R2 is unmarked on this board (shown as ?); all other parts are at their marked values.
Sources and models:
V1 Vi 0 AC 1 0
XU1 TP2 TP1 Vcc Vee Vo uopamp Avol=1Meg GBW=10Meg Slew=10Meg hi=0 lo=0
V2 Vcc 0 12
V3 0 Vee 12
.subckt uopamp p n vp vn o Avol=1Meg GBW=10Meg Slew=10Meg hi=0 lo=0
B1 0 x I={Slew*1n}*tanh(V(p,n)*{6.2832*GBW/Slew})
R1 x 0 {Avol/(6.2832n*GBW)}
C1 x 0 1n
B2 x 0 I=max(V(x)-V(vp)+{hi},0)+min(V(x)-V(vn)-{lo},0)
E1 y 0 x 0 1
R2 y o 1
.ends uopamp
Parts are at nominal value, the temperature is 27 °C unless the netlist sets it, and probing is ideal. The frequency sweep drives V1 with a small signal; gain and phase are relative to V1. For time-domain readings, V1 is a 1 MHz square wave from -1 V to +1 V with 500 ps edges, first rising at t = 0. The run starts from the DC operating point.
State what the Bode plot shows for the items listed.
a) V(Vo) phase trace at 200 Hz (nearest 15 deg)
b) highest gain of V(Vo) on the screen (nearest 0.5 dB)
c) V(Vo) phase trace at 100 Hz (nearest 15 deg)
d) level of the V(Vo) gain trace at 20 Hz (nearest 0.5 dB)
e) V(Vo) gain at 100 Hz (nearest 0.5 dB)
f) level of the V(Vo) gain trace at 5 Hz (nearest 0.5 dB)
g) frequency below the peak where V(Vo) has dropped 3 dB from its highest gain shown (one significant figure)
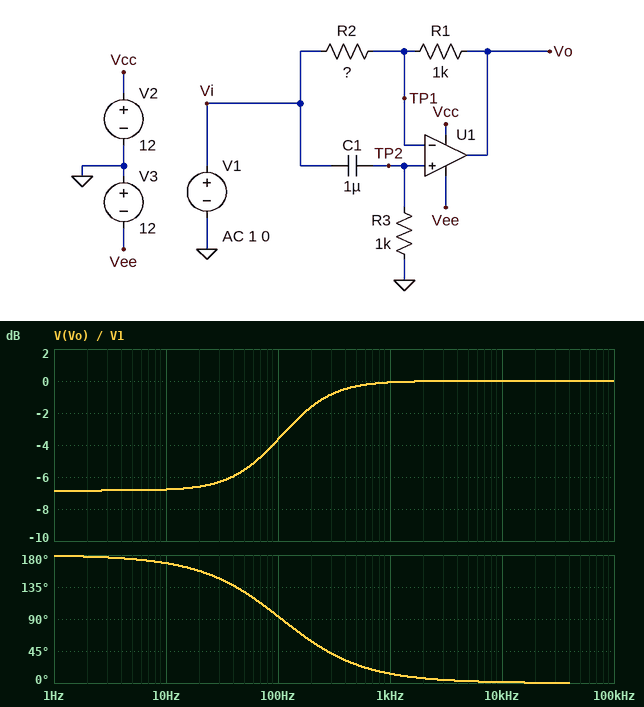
60 deg
0 dB
90 deg
-6.5 dB
-3.5 dB
-7.0 dB
100 Hz
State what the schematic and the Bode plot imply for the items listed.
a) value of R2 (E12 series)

2.2 kΩ
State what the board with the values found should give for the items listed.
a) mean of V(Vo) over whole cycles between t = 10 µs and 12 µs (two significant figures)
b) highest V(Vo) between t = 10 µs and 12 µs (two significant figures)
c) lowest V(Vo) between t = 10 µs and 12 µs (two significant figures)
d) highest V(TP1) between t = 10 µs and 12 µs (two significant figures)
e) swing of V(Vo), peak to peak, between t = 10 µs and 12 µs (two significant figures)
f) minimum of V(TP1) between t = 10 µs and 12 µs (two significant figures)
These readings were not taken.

1.4 V
2.4 V
440 mV
2.0 V
2.0 V
-12 mV
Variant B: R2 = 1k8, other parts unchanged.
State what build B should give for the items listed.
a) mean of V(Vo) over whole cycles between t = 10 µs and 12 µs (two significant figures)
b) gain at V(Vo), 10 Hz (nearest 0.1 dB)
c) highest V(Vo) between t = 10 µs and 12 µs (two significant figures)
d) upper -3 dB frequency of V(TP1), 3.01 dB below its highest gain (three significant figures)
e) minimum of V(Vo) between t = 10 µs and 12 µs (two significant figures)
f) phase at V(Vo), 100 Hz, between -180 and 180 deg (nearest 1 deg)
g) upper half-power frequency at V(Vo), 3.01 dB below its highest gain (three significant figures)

1.5 V
-5.1 dB
2.5 V
7.45 MHz
540 mV
99 deg
6.43 MHz
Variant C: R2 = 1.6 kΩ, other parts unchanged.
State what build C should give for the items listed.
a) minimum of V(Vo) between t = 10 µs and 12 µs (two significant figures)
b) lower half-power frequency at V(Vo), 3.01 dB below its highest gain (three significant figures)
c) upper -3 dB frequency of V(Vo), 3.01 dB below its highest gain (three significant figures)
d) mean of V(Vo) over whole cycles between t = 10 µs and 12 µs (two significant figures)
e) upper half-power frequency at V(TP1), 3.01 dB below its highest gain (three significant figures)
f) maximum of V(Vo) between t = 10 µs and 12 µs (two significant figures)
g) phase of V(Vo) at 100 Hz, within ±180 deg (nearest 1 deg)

610 mV
74.4 Hz
6.15 MHz
1.6 V
7.33 MHz
2.6 V
103 deg
